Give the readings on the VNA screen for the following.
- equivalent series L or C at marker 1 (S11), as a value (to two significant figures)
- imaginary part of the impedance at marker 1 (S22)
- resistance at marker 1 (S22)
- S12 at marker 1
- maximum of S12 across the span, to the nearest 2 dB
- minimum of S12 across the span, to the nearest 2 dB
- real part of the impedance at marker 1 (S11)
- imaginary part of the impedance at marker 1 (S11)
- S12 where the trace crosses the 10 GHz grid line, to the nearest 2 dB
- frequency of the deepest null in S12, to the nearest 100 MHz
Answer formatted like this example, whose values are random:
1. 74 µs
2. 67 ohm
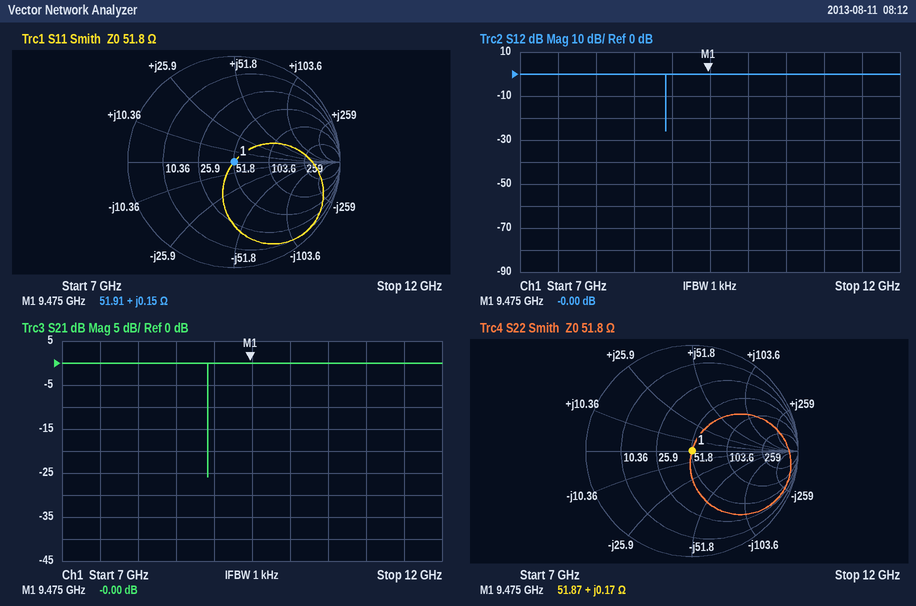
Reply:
1. 2.5 pH
2. +0.17 Ω
3. 51.87 Ω
4. -0.00 dB
5. 0 dB
6. -26 dB
7. 51.91 Ω
8. +0.15 Ω
9. 0 dB
10. 8.9 GHz
